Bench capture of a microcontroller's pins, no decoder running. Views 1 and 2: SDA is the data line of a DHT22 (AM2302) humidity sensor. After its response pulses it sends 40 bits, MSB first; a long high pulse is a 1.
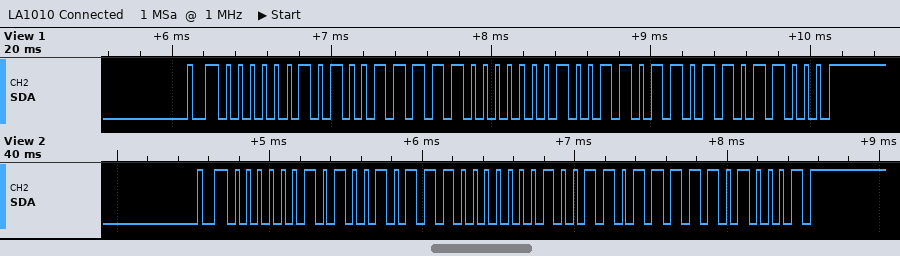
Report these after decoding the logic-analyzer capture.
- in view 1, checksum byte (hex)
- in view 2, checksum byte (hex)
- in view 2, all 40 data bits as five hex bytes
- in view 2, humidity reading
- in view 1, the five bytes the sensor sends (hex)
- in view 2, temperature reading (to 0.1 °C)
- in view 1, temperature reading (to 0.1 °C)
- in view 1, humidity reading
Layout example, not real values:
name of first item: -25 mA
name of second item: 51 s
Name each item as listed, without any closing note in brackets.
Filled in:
in view 1, checksum byte: 0xD8
in view 2, checksum byte: 0xD1
in view 2, all 40 data bits as five hex bytes: 02 97 01 37 D1
in view 2, humidity reading: 66.3 %
in view 1, the five bytes the sensor sends: 02 9F 01 36 D8
in view 2, temperature reading: 31.1 °C
in view 1, temperature reading: 31.0 °C
in view 1, humidity reading: 67.1 %
